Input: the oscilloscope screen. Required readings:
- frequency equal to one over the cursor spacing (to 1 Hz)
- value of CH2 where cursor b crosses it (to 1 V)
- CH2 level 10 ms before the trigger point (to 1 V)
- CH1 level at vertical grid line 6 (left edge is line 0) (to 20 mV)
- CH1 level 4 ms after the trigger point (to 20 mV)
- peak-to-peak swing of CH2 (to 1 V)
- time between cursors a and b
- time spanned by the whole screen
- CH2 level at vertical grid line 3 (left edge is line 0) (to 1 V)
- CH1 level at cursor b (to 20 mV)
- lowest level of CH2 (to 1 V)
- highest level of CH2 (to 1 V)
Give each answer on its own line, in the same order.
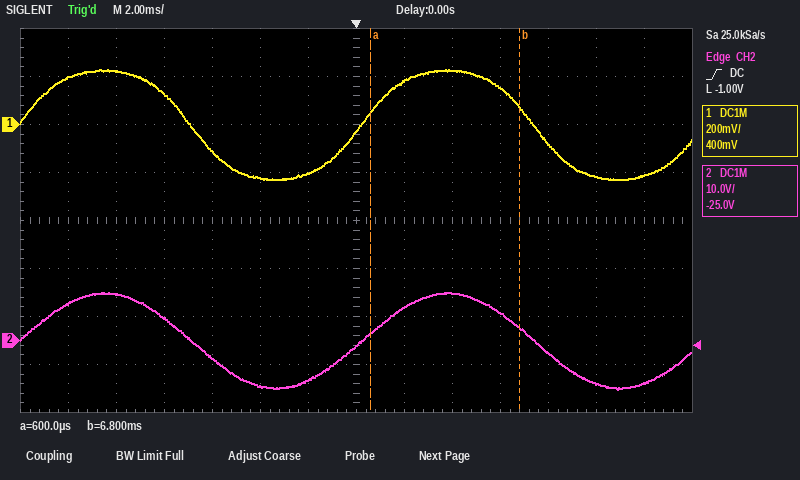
161 Hz
3 V
10 V
-200 mV
220 mV
20 V
6.2 ms
28 ms
5 V
80 mV
-10 V
10 V
